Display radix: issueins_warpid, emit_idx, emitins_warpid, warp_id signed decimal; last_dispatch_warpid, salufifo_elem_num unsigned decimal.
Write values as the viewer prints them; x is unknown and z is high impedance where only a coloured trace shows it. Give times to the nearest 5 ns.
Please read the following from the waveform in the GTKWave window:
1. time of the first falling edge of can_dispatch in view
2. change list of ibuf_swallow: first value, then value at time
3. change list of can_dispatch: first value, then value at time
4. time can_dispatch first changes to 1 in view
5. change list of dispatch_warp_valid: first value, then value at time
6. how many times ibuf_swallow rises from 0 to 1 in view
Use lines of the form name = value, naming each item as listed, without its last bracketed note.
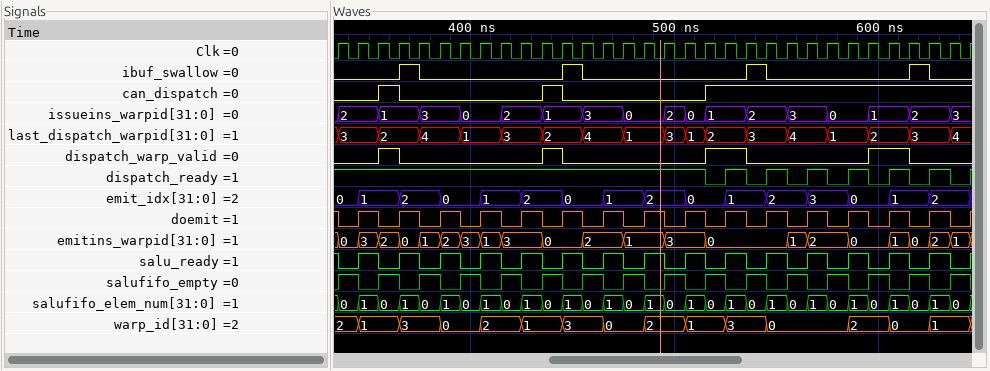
time of the first falling edge of can_dispatch in view = 365 ns
change list of ibuf_swallow: first value, then value at time = 0, 1 at 365 ns, 0 at 375 ns, 1 at 445 ns, 0 at 455 ns, 1 at 535 ns, 0 at 545 ns, 1 at 615 ns, 0 at 625 ns
change list of can_dispatch: first value, then value at time = 0, 1 at 355 ns, 0 at 365 ns, 1 at 435 ns, 0 at 445 ns, 1 at 515 ns
time can_dispatch first changes to 1 in view = 355 ns
change list of dispatch_warp_valid: first value, then value at time = 0, 1 at 355 ns, 0 at 365 ns, 1 at 435 ns, 0 at 445 ns, 1 at 515 ns, 0 at 535 ns, 1 at 595 ns, 0 at 615 ns
how many times ibuf_swallow rises from 0 to 1 in view = 4
